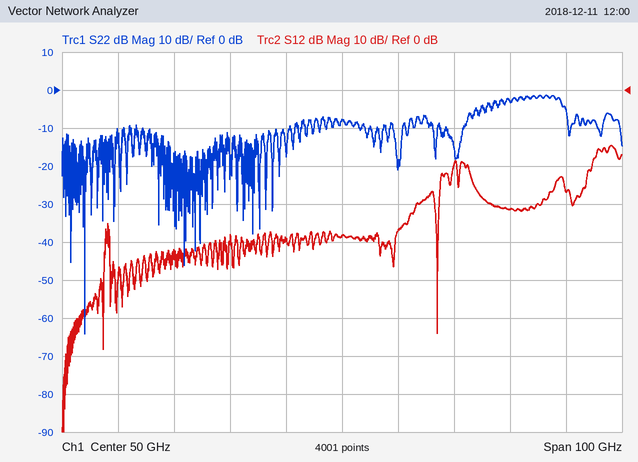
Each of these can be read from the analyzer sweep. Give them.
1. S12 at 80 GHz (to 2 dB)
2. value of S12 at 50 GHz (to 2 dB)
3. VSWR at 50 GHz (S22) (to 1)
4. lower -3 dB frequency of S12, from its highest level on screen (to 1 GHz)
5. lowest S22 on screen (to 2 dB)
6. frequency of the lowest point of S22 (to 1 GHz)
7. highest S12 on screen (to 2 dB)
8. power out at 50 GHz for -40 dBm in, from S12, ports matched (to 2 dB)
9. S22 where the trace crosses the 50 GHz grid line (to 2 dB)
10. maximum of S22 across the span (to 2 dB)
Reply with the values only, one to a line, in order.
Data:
-32 dB
-38 dB
2
95 GHz
-64 dB
4 GHz
-14 dB
-78 dBm
-8 dB
-2 dB
